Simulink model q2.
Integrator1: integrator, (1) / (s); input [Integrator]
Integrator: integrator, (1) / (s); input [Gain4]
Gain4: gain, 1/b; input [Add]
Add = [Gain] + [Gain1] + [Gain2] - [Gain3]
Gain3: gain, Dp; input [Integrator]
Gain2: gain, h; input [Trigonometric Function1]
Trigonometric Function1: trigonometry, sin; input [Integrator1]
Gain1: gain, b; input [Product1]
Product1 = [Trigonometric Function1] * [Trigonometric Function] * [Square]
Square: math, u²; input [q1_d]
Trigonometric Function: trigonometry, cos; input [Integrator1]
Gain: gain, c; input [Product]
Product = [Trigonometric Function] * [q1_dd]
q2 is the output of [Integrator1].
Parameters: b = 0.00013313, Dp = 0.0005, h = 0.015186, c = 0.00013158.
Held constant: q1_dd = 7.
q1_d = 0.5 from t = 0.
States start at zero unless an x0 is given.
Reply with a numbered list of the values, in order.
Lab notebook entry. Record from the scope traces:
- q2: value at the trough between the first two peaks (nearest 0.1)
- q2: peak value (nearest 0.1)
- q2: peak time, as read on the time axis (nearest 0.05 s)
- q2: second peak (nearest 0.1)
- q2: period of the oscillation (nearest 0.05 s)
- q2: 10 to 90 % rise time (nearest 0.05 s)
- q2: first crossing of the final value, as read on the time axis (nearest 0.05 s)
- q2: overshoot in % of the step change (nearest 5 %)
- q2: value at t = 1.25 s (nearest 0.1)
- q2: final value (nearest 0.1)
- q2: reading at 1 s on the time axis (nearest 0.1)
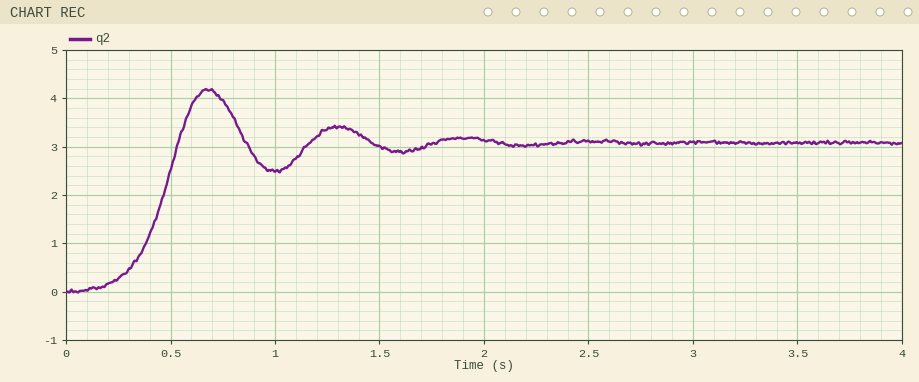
1. 2.5
2. 4.2
3. 0.70 s
4. 3.4
5. 0.60 s
6. 0.25 s
7. 0.55 s
8. 35 %
9. 3.4
10. 3.1
11. 2.5
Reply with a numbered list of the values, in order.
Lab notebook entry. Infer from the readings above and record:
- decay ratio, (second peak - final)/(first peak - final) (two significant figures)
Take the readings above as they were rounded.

1. 0.27
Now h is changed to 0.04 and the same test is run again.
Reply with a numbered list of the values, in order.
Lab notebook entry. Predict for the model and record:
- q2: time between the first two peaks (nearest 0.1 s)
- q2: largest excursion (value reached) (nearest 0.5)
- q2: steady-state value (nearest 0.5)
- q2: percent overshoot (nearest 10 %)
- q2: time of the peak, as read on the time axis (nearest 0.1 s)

1. 0.4 s
2. 4.5
3. 3.0
4. 50 %
5. 0.5 s
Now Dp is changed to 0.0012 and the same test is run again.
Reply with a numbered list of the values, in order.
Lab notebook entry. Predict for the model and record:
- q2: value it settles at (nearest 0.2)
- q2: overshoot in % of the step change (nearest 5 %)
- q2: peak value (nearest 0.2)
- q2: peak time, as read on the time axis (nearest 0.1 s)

1. 3.0
2. 10 %
3. 3.4
4. 0.8 s
